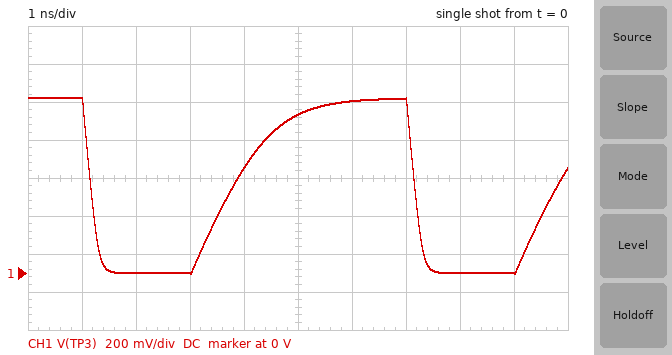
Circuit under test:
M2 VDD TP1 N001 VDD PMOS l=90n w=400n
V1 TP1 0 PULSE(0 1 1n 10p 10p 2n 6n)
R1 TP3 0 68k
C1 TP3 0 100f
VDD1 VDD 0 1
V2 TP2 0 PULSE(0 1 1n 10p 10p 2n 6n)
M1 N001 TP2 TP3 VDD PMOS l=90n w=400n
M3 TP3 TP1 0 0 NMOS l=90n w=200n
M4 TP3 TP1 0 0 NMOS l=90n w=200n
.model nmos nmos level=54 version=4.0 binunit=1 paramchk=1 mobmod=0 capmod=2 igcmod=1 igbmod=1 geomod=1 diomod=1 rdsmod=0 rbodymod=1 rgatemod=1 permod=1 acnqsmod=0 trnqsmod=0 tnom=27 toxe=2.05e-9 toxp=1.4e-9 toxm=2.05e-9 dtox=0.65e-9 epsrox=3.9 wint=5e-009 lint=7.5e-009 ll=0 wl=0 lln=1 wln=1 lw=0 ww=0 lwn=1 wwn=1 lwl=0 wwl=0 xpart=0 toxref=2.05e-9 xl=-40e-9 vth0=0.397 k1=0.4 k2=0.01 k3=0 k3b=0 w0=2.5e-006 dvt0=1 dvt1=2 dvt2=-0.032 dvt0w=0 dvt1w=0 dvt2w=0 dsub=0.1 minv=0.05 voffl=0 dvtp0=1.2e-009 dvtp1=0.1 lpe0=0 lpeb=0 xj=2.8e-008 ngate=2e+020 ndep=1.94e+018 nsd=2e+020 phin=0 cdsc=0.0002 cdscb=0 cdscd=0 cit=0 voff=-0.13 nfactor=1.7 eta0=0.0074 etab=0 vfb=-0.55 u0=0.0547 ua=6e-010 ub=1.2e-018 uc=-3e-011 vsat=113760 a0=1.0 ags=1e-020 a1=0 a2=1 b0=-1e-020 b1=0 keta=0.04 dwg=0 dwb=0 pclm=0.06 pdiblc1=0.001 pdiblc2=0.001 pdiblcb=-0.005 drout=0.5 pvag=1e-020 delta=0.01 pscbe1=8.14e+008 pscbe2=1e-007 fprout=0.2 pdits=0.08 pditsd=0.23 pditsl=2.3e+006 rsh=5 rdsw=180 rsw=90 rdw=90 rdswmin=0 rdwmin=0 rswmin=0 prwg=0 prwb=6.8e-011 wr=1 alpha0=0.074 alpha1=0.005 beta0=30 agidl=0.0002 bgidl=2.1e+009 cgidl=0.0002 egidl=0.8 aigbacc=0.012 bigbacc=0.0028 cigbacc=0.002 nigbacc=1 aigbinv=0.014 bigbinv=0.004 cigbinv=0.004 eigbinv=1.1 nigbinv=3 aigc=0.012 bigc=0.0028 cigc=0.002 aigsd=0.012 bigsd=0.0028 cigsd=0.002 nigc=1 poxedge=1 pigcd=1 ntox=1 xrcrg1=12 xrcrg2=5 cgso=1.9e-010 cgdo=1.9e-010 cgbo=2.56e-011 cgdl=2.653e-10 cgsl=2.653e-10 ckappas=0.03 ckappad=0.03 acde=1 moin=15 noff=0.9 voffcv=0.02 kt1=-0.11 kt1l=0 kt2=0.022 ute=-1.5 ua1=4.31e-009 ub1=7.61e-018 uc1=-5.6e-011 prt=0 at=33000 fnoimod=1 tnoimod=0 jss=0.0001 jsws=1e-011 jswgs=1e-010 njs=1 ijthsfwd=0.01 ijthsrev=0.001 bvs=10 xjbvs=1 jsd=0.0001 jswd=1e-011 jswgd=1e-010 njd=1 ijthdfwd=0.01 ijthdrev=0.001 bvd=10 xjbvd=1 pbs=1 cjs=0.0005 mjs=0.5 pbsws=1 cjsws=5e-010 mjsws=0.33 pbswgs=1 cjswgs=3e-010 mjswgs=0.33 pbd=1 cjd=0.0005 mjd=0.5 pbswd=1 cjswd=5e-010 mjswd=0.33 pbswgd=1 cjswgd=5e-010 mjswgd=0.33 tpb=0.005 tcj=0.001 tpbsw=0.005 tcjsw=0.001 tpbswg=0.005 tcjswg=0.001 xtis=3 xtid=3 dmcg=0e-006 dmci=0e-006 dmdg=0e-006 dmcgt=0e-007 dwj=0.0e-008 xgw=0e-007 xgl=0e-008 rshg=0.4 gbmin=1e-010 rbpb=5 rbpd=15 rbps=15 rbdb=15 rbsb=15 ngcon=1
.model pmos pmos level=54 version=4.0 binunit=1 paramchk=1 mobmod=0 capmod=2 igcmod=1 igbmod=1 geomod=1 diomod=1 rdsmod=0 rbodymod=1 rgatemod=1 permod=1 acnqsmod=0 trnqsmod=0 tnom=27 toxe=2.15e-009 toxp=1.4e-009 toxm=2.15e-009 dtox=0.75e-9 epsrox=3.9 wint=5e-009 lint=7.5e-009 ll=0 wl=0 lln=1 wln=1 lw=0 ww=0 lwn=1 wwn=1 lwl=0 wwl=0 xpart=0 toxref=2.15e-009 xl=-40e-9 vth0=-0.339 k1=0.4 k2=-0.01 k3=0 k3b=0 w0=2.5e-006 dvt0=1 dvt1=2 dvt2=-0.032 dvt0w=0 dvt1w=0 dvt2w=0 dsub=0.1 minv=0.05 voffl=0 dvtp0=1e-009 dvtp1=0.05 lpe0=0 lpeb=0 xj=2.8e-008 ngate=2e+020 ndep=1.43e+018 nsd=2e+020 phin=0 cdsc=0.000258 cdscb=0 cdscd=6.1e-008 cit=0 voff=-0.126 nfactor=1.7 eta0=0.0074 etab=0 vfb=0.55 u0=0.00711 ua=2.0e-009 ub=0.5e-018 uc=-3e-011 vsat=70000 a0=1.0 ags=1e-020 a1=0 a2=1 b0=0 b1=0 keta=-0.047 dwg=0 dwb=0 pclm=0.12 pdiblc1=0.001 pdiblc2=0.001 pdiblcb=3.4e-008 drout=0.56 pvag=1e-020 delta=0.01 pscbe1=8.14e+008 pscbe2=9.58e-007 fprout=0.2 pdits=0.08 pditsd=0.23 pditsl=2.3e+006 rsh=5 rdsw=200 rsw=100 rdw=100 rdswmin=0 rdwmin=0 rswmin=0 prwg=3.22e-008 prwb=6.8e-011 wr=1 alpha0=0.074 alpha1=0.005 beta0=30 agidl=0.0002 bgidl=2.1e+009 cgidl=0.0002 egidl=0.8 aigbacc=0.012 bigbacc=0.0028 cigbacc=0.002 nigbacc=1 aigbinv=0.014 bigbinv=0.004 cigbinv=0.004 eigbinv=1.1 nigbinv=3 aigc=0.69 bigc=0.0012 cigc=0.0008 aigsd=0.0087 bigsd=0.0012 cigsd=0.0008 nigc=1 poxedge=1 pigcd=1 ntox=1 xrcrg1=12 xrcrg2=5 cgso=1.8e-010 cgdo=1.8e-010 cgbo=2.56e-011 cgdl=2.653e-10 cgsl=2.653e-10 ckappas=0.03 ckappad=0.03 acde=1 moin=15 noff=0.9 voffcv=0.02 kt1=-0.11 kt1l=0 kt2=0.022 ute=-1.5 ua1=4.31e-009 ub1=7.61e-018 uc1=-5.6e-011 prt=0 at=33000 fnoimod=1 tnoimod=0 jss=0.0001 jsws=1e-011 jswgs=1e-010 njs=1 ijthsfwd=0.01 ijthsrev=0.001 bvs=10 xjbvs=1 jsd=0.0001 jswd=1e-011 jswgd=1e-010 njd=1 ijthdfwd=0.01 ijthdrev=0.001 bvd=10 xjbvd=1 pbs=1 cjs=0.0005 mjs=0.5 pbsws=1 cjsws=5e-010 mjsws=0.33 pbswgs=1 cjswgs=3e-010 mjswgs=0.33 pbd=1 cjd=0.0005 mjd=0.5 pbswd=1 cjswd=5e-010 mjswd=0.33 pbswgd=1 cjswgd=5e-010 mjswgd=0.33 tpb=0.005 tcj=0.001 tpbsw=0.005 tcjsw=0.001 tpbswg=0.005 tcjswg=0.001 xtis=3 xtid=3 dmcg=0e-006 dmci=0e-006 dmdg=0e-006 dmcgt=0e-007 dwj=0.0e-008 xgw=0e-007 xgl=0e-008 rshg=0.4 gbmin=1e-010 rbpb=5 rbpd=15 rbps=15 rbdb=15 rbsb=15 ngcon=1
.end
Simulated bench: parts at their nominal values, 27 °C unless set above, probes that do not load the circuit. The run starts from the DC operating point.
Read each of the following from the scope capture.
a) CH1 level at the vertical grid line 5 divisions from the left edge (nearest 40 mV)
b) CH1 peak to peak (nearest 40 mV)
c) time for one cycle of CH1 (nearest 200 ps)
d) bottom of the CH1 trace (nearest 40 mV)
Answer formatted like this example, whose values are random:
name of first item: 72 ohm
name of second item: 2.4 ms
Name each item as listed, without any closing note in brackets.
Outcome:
CH1 level at the vertical grid line 5 divisions from the left edge: 840 mV
CH1 peak to peak: 920 mV
time for one cycle of CH1: 6.0 ns
bottom of the CH1 trace: 0 V
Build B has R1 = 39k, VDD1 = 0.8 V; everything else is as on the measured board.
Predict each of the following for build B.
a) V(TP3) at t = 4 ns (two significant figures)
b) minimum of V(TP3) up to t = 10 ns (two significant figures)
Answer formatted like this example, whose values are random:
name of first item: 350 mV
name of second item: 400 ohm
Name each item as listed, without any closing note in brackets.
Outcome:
V(TP3) at t = 4 ns: 310 mV
minimum of V(TP3) up to t = 10 ns: -3.7 mV
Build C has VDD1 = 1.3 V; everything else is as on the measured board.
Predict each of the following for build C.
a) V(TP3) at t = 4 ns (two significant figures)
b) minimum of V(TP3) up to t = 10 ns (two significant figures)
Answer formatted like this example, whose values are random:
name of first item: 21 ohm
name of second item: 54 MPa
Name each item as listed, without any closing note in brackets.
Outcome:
V(TP3) at t = 4 ns: 890 mV
minimum of V(TP3) up to t = 10 ns: -1.7 mV
